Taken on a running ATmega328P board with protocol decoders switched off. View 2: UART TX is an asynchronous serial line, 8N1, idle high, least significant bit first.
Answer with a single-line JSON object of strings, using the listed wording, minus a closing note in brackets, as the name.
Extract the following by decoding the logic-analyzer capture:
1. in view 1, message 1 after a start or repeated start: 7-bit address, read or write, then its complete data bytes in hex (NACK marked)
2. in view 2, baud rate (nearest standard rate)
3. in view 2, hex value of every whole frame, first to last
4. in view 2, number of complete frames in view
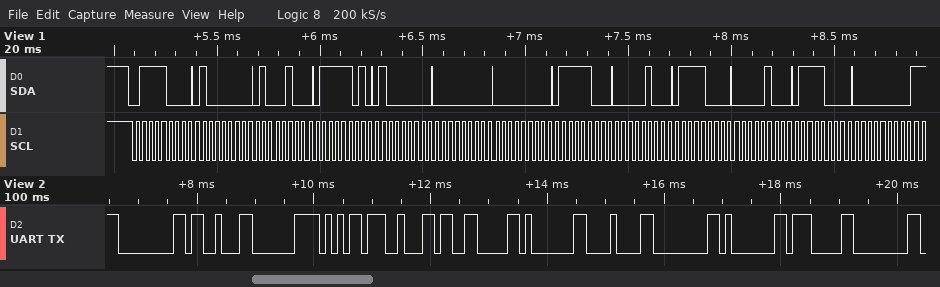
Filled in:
{"in view 1, message 1 after a start or repeated start: 7-bit address, read or write, then its complete data bytes in hex": "0x3C write: 40 44 7D 40 00 00 7C 04 78 04 78 00", "in view 2, baud rate": "9600 baud", "in view 2, hex value of every whole frame, first to last": "00 13 C0 B5 62 06 01 08 00 01 07 00", "in view 2, number of complete frames in view": "12"}
